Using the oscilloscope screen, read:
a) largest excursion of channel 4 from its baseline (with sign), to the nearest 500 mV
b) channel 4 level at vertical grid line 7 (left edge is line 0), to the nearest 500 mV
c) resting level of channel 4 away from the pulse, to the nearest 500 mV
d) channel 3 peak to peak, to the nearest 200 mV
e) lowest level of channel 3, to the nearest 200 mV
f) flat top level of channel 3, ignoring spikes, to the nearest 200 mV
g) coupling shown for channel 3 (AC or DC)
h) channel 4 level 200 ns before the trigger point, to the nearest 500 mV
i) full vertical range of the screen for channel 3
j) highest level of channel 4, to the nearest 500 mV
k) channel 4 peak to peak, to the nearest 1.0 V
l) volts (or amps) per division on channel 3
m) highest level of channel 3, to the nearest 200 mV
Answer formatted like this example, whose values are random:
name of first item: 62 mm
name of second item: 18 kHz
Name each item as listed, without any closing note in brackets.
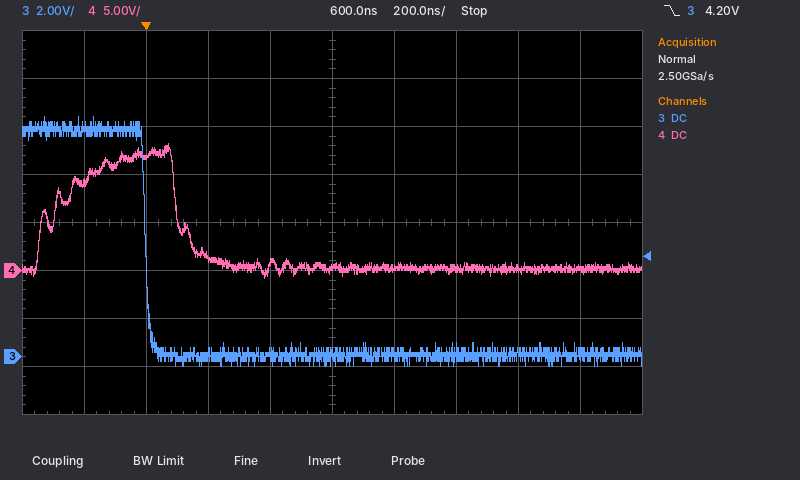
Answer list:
largest excursion of channel 4 from its baseline (with sign), to the nearest 500 mV: +13.0 V
channel 4 level at vertical grid line 7 (left edge is line 0), to the nearest 500 mV: 0.0 V
resting level of channel 4 away from the pulse, to the nearest 500 mV: 0.0 V
channel 3 peak to peak, to the nearest 200 mV: 10.4 V
lowest level of channel 3, to the nearest 200 mV: -400 mV
flat top level of channel 3, ignoring spikes, to the nearest 200 mV: 9.4 V
coupling shown for channel 3: DC
channel 4 level 200 ns before the trigger point, to the nearest 500 mV: 9.0 V
full vertical range of the screen for channel 3: 16 V
highest level of channel 4, to the nearest 500 mV: 13.0 V
channel 4 peak to peak, to the nearest 1.0 V: 14.0 V
volts (or amps) per division on channel 3: 2 V
highest level of channel 3, to the nearest 200 mV: 10.0 V
